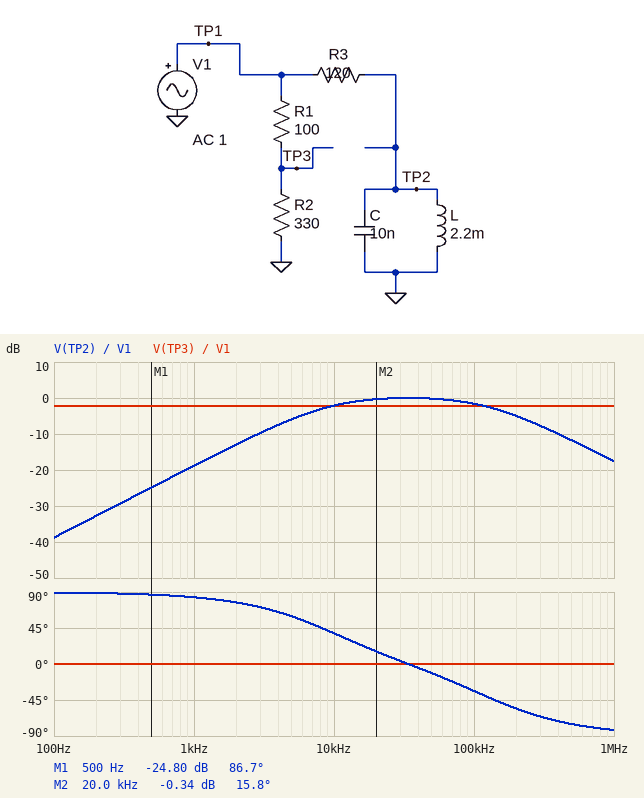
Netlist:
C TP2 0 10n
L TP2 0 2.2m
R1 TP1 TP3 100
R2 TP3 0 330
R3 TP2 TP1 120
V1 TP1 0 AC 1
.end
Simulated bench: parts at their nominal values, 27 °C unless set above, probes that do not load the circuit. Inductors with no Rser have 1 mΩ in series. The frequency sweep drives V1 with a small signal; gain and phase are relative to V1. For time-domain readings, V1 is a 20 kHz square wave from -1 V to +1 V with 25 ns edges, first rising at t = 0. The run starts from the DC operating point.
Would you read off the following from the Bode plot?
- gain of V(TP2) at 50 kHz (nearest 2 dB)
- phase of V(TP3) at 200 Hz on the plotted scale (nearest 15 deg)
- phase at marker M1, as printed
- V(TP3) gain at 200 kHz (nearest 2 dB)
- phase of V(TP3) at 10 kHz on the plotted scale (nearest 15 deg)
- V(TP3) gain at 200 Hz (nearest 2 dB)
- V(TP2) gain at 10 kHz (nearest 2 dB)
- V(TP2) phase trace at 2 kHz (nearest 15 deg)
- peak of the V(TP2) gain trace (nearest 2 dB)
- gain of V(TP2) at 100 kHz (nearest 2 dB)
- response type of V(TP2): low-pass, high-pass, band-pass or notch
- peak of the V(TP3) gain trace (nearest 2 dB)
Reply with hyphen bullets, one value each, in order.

- 0 dB
- 0 deg
- 86.7 deg
- -2 dB
- 0 deg
- -2 dB
- -2 dB
- 75 deg
- 0 dB
- -2 dB
- band-pass
- -2 dB
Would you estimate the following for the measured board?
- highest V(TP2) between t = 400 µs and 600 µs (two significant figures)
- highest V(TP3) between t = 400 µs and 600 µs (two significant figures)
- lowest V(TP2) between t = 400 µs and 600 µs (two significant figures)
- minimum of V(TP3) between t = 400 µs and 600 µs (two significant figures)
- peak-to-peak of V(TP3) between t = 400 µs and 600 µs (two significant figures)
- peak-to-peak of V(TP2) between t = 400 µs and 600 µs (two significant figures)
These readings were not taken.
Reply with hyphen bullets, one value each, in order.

- 1.4 V
- 770 mV
- -1.4 V
- -770 mV
- 1.5 V
- 2.8 V
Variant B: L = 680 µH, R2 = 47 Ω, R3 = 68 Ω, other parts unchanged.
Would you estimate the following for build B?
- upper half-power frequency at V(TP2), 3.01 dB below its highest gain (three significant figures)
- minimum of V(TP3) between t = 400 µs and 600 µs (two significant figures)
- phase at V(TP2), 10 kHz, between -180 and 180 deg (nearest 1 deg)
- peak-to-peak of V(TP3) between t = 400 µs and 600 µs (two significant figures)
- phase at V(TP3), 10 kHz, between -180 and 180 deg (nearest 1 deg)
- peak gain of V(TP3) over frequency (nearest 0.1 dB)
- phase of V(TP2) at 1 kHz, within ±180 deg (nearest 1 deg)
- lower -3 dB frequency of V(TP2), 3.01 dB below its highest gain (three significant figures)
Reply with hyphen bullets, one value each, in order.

- 249 kHz
- -320 mV
- 57 deg
- 640 mV
- 0 deg
- -9.9 dB
- 86 deg
- 15.0 kHz
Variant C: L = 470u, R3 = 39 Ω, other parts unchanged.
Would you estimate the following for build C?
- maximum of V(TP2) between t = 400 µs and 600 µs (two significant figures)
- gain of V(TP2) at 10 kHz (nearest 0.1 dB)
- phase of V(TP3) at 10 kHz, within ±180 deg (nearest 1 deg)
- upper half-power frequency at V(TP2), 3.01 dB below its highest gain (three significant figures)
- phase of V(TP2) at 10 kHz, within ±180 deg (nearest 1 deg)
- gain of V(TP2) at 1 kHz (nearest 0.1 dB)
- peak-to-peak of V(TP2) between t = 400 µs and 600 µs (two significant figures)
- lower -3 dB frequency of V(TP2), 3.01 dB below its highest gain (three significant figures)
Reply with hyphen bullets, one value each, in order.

- 1.6 V
- -4.3 dB
- 0 deg
- 421 kHz
- 52 deg
- -22.4 dB
- 3.3 V
- 12.8 kHz
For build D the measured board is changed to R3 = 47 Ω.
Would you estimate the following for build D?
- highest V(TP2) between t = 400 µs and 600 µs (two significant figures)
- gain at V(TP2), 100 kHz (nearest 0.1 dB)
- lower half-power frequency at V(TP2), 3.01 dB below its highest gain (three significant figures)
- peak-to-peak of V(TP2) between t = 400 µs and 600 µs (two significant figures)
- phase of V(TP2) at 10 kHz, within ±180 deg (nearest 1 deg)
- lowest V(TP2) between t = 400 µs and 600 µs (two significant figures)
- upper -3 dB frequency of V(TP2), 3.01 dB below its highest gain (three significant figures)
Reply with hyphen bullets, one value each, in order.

- 1.2 V
- -0.3 dB
- 3.37 kHz
- 2.4 V
- 17 deg
- -1.2 V
- 342 kHz
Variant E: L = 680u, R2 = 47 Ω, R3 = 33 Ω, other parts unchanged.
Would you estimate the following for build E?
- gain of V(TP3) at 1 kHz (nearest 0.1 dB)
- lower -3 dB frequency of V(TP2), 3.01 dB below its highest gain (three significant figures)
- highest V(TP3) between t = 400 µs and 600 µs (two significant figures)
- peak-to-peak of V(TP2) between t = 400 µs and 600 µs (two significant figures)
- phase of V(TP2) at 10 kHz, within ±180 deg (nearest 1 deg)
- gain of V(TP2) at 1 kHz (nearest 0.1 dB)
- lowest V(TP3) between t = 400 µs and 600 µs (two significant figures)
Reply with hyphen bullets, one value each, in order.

- -9.9 dB
- 7.60 kHz
- 320 mV
- 2.9 V
- 37 deg
- -17.8 dB
- -320 mV
